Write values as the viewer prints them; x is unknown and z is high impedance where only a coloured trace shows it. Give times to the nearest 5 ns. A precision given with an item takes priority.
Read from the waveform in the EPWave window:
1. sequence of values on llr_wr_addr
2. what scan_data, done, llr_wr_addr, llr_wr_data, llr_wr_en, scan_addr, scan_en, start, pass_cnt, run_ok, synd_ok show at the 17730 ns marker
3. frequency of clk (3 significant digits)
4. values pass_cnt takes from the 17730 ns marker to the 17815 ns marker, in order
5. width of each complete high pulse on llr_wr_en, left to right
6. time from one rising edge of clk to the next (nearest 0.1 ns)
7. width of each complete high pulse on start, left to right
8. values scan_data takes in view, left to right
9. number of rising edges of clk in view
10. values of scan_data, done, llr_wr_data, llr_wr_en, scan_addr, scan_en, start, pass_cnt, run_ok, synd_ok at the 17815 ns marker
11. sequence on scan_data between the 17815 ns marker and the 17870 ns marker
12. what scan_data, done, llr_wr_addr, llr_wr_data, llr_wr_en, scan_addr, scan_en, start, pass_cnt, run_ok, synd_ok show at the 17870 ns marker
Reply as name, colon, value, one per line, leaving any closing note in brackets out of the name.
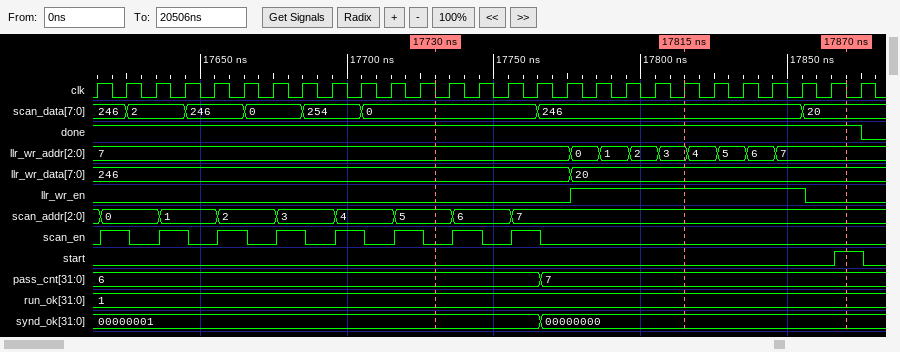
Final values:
sequence of values on llr_wr_addr: 7, 0, 1, 2, 3, 4, 5, 6, 7
what scan_data, done, llr_wr_addr, llr_wr_data, llr_wr_en, scan_addr, scan_en, start, pass_cnt, run_ok, synd_ok show at the 17730 ns marker: scan_data=0, done=1, llr_wr_addr=7, llr_wr_data=246, llr_wr_en=0, scan_addr=5, scan_en=0, start=0, pass_cnt=6, run_ok=1, synd_ok=00000001
frequency of clk: 100 MHz
values pass_cnt takes from the 17730 ns marker to the 17815 ns marker, in order: 6, 7
width of each complete high pulse on llr_wr_en, left to right: 80 ns
time from one rising edge of clk to the next: 10 ns
width of each complete high pulse on start, left to right: 10 ns
values scan_data takes in view, left to right: 246, 2, 246, 0, 254, 0, 246, 20
number of rising edges of clk in view: 27
values of scan_data, done, llr_wr_data, llr_wr_en, scan_addr, scan_en, start, pass_cnt, run_ok, synd_ok at the 17815 ns marker: scan_data=246, done=1, llr_wr_data=20, llr_wr_en=1, scan_addr=7, scan_en=0, start=0, pass_cnt=7, run_ok=1, synd_ok=00000000
sequence on scan_data between the 17815 ns marker and the 17870 ns marker: 246, 20
what scan_data, done, llr_wr_addr, llr_wr_data, llr_wr_en, scan_addr, scan_en, start, pass_cnt, run_ok, synd_ok show at the 17870 ns marker: scan_data=20, done=1, llr_wr_addr=7, llr_wr_data=20, llr_wr_en=0, scan_addr=7, scan_en=0, start=1, pass_cnt=7, run_ok=1, synd_ok=00000000
